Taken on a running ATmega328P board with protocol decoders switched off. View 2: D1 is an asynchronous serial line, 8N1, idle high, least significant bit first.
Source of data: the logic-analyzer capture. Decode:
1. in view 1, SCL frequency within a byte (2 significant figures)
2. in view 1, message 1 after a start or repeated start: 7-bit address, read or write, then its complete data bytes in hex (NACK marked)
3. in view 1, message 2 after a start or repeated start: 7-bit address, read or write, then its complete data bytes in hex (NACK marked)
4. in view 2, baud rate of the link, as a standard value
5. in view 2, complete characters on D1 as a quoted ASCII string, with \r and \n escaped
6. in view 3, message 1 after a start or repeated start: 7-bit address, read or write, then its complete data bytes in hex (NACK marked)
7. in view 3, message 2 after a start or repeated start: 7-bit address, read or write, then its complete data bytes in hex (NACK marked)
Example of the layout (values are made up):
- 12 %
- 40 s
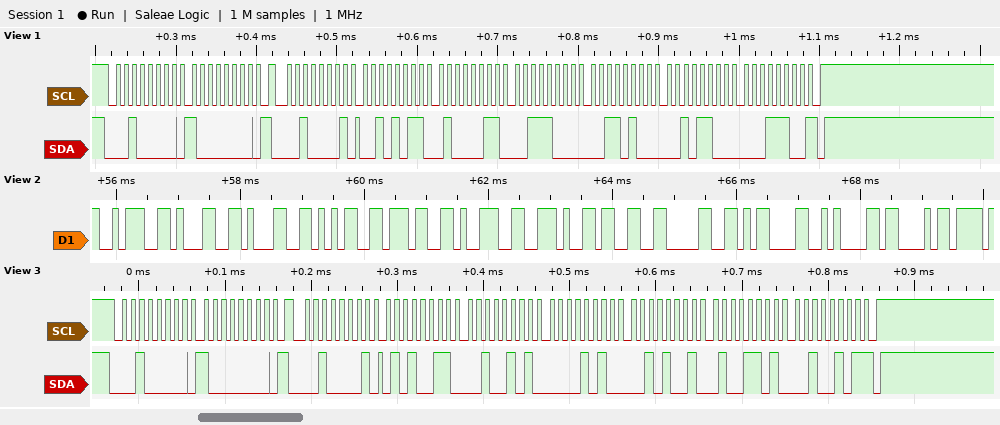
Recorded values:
- 100 kHz
- 0x10 write: 80
- 0x10 read: 2B 43 38 34 2C 1C NACK
- 9600 baud
- ":11579.30\r\nC"
- 0x10 write: 80
- 0x10 read: 53 25 0A 29 4D 25 NACK
